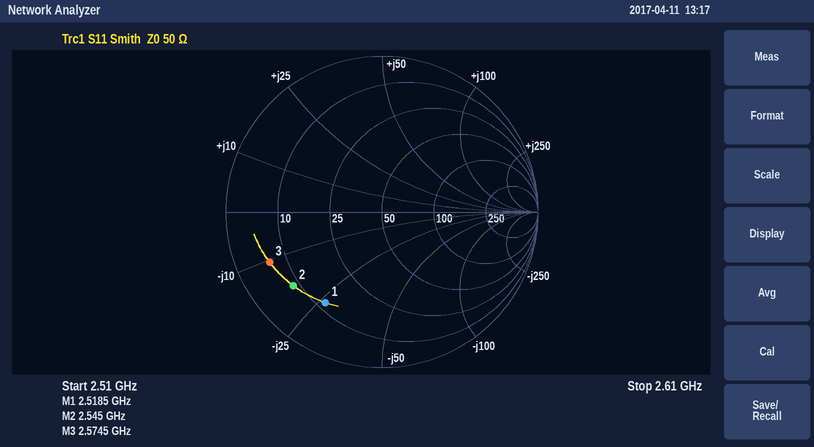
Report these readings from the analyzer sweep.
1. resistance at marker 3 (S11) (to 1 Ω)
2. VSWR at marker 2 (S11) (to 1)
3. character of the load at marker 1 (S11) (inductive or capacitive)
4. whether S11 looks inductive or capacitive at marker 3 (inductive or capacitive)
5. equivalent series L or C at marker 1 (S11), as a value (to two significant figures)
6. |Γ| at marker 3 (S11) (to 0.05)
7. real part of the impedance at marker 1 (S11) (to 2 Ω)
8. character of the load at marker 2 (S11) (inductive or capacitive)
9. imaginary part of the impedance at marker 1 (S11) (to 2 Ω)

6 Ω
7
capacitive
capacitive
2.4 pF
0.80
12 Ω
capacitive
-26 Ω
